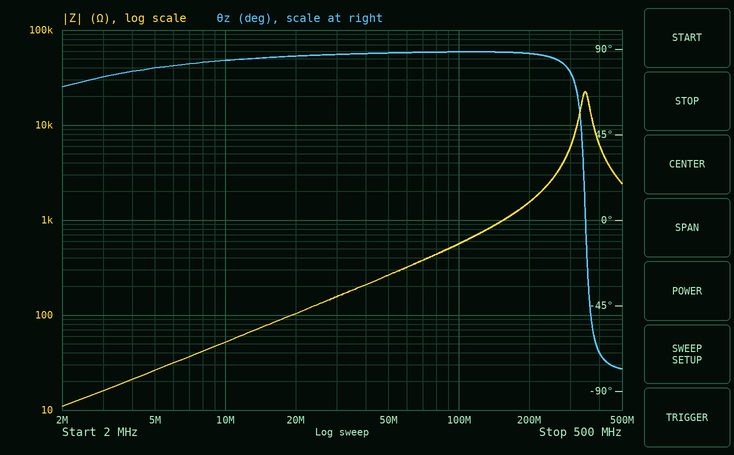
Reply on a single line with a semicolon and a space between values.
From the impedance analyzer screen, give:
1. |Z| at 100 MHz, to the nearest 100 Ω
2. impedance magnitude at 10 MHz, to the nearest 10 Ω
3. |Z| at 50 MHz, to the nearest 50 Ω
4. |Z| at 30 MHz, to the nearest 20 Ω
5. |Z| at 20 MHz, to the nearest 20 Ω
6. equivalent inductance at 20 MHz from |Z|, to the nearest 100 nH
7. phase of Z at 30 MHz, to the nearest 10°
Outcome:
600 Ω; 50 Ω; 250 Ω; 160 Ω; 100 Ω; 800 nH; 90°
